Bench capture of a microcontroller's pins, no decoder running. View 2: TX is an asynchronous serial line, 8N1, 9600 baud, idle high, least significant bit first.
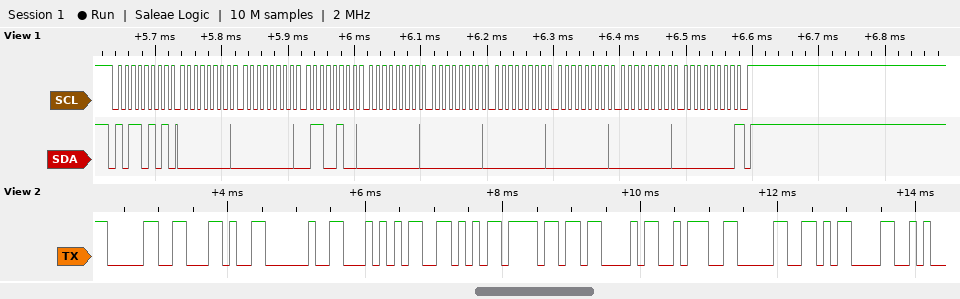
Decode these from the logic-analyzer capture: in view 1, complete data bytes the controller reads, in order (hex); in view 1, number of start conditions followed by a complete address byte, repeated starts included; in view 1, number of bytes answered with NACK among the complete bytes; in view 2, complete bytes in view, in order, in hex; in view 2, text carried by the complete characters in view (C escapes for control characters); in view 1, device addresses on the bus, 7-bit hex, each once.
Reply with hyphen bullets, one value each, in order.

- 00 00 64 00 00 00 00 00 00
- 1
- 1
- 30 2C 20 54 56 6F 43 3A 30 0D
- "0, TVoC:0\r"
- 0x5A
